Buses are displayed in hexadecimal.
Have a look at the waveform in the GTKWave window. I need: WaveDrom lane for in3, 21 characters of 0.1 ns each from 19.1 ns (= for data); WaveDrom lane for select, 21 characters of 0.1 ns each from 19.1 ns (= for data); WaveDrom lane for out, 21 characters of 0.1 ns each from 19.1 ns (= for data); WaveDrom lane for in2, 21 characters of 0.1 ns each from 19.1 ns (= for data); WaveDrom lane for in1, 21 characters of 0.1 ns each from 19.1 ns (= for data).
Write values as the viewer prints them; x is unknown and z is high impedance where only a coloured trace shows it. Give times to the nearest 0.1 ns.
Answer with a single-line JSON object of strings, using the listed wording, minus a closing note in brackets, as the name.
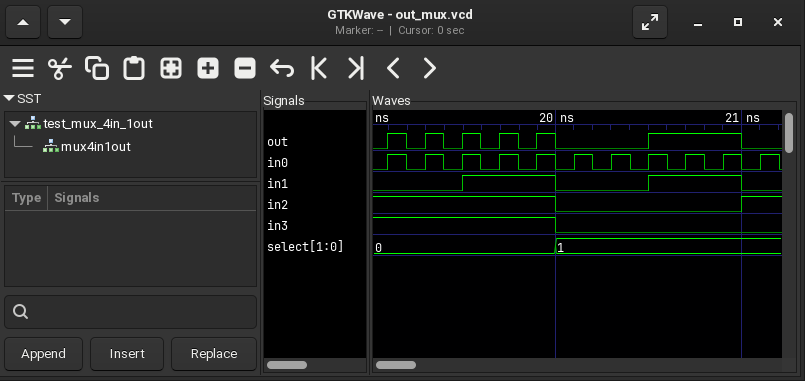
{"WaveDrom lane for in3, 21 characters of 0.1 ns each from 19.1 ns": "{name: 'in3', wave: '1........0...........'}", "WaveDrom lane for select, 21 characters of 0.1 ns each from 19.1 ns": "{name: 'select', wave: '=........=...........', data: '0 1'}", "WaveDrom lane for out, 21 characters of 0.1 ns each from 19.1 ns": "{name: 'out', wave: '1010101010....1....0.'}", "WaveDrom lane for in2, 21 characters of 0.1 ns each from 19.1 ns": "{name: 'in2', wave: '1........0.........1.'}", "WaveDrom lane for in1, 21 characters of 0.1 ns each from 19.1 ns": "{name: 'in1', wave: '0...1....0....1....0.'}"}
